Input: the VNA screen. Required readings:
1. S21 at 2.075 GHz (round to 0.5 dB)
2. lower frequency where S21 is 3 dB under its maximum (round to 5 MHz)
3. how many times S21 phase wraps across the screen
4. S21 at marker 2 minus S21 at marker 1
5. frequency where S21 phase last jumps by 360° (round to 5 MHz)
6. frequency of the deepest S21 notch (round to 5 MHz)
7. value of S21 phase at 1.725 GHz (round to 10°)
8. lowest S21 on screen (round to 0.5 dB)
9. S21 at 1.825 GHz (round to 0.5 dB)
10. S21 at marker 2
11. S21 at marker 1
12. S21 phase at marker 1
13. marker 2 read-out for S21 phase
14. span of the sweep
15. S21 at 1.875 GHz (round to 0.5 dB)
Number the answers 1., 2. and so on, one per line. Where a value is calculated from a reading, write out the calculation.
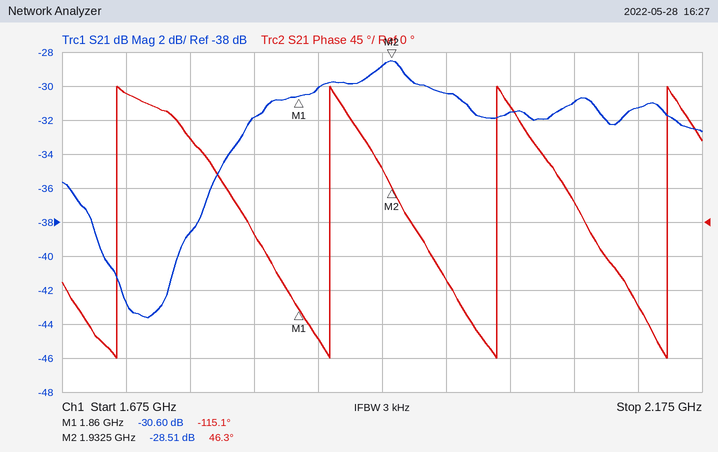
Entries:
1. -31.0 dB
2. 1.830 GHz
3. 4
4. -28.51 − (-30.6) = 2.09 dB
5. 2.150 GHz
6. 1.740 GHz
7. 170°
8. -43.5 dB
9. -32.0 dB
10. -28.51 dB
11. -30.60 dB
12. -115.1°
13. 46.3°
14. 500 MHz
15. -30.0 dB
